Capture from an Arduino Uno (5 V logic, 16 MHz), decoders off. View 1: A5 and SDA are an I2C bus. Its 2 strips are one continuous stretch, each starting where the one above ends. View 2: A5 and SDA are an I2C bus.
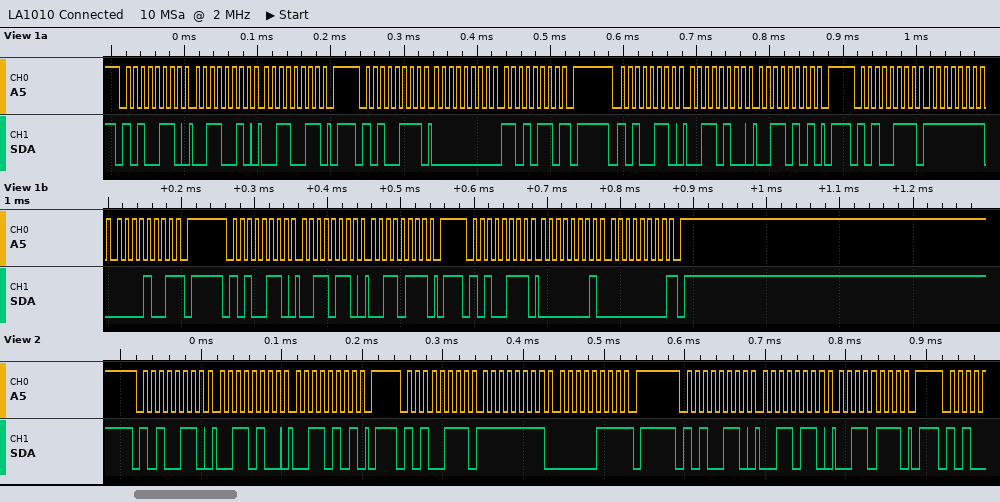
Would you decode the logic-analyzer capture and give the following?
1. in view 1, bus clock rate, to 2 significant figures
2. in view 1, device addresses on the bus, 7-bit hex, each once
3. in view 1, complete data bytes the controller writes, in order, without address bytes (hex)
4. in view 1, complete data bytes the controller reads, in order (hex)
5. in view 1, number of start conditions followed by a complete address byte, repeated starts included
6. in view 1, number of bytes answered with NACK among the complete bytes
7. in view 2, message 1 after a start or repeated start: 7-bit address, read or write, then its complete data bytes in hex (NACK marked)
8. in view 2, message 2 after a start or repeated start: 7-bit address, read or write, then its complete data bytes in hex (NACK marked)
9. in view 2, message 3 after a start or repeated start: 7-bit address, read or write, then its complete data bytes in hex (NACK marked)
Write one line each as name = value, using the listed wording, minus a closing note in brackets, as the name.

in view 1, bus clock rate, to 2 significant figures = 100 kHz
in view 1, device addresses on the bus, 7-bit hex, each once = 0x53
in view 1, complete data bytes the controller writes, in order, without address bytes = 32 33 34 35 36 37
in view 1, complete data bytes the controller reads, in order = 00 D6 FF 09 01 00
in view 1, number of start conditions followed by a complete address byte, repeated starts included = 6
in view 1, number of bytes answered with NACK among the complete bytes = 3
in view 2, message 1 after a start or repeated start: 7-bit address, read or write, then its complete data bytes in hex = 0x53 write: 34 35
in view 2, message 2 after a start or repeated start: 7-bit address, read or write, then its complete data bytes in hex = 0x53 read: FF 07 NACK
in view 2, message 3 after a start or repeated start: 7-bit address, read or write, then its complete data bytes in hex = 0x53 write: 36 37
